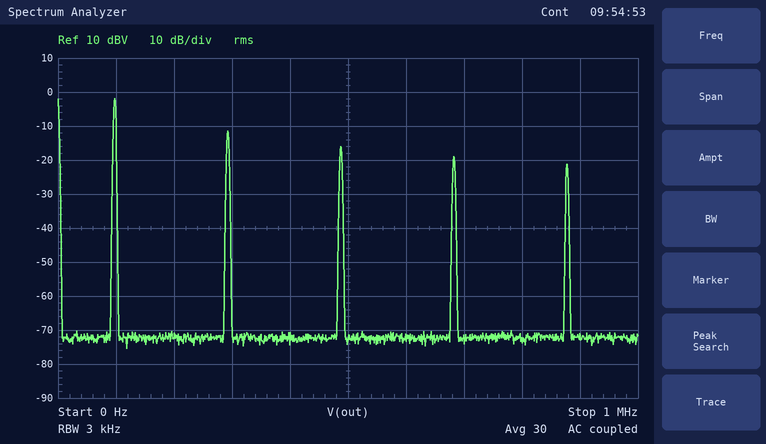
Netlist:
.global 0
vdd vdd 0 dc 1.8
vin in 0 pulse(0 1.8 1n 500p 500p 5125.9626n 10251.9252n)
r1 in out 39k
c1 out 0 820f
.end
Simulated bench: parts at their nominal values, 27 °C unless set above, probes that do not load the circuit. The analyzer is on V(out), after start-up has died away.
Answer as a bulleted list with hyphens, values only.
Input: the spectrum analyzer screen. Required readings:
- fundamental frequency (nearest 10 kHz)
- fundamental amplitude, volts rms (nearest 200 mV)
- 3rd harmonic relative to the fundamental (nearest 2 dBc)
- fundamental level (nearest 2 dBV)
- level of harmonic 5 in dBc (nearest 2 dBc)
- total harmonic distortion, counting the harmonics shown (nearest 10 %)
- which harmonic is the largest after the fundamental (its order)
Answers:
- 100 kHz
- 800 mV
- -10 dBc
- -2 dBV
- -14 dBc
- 40 %
- 3
